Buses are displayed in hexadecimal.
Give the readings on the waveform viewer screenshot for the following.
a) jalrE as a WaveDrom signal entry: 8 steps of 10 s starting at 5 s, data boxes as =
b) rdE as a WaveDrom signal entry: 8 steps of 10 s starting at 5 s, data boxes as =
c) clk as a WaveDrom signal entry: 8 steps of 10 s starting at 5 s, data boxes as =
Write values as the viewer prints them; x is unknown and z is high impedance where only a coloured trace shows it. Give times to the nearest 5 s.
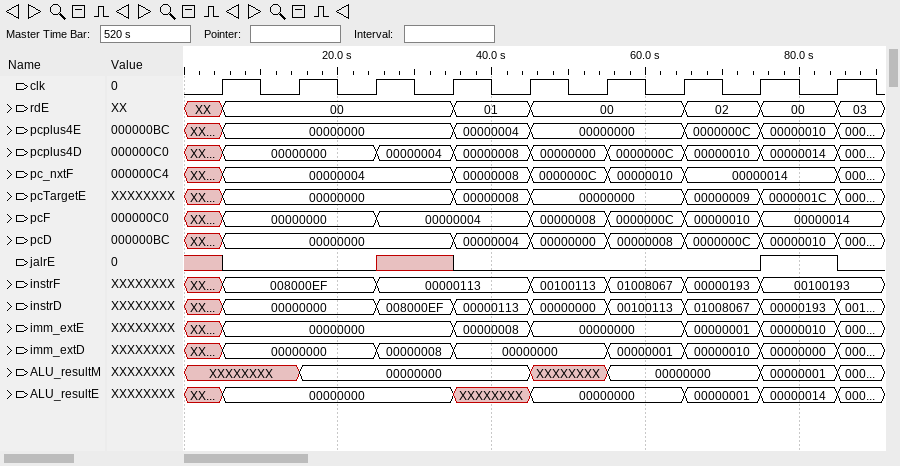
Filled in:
{name: 'jalrE', wave: '0.x0...1'}
{name: 'rdE', wave: '=..==.==', data: '00 01 00 02 00'}
{name: 'clk', wave: 'p.......'}
